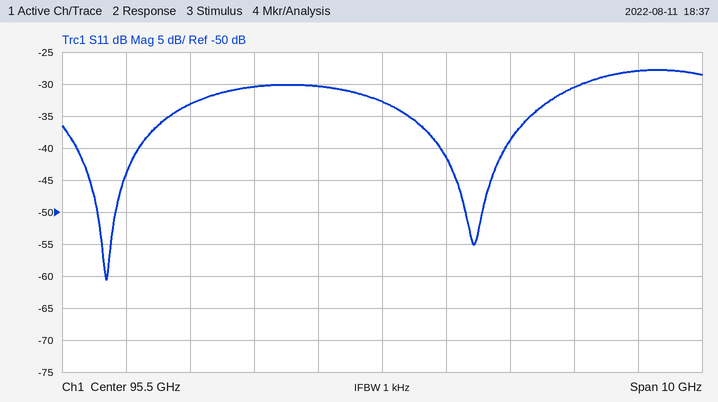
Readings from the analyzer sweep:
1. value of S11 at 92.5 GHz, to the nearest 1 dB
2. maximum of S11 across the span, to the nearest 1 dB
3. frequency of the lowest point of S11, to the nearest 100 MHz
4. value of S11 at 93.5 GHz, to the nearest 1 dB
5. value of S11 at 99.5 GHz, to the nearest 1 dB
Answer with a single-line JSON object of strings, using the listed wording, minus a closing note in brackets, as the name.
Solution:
{"value of S11 at 92.5 GHz, to the nearest 1 dB": "-33 dB", "maximum of S11 across the span, to the nearest 1 dB": "-28 dB", "frequency of the lowest point of S11, to the nearest 100 MHz": "91.2 GHz", "value of S11 at 93.5 GHz, to the nearest 1 dB": "-30 dB", "value of S11 at 99.5 GHz, to the nearest 1 dB": "-28 dB"}
